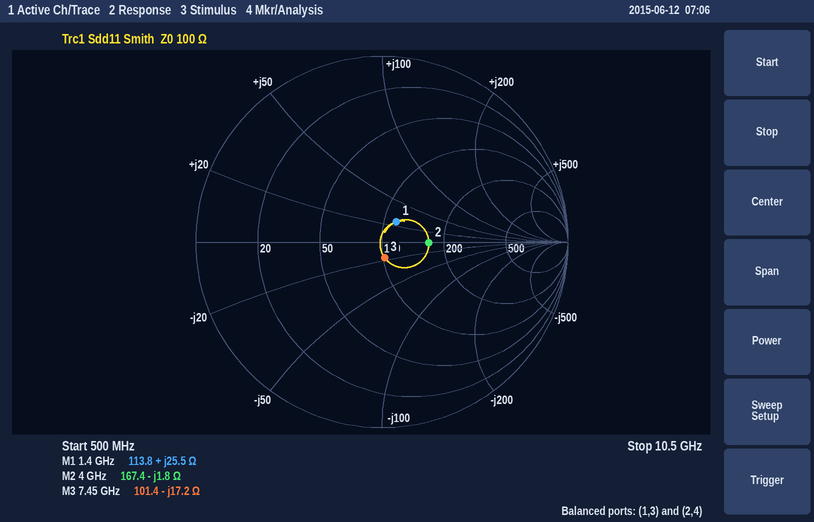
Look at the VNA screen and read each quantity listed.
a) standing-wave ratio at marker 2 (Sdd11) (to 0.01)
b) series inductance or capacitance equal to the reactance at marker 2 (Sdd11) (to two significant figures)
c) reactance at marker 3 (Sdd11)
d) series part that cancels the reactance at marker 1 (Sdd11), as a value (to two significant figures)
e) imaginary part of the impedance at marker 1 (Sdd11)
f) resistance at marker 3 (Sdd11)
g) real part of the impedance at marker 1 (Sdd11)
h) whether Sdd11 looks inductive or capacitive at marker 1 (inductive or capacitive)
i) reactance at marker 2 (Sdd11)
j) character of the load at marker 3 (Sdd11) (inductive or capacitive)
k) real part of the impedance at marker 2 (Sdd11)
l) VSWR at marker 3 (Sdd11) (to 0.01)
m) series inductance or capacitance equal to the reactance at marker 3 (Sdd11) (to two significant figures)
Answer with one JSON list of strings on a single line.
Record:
["1.67", "22 pF", "-17.2 Ω", "4.5 pF", "+25.5 Ω", "101.4 Ω", "113.8 Ω", "inductive", "-1.8 Ω", "capacitive", "167.4 Ω", "1.19", "1.2 pF"]
